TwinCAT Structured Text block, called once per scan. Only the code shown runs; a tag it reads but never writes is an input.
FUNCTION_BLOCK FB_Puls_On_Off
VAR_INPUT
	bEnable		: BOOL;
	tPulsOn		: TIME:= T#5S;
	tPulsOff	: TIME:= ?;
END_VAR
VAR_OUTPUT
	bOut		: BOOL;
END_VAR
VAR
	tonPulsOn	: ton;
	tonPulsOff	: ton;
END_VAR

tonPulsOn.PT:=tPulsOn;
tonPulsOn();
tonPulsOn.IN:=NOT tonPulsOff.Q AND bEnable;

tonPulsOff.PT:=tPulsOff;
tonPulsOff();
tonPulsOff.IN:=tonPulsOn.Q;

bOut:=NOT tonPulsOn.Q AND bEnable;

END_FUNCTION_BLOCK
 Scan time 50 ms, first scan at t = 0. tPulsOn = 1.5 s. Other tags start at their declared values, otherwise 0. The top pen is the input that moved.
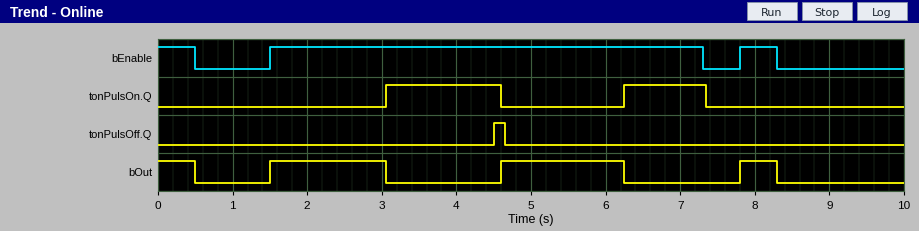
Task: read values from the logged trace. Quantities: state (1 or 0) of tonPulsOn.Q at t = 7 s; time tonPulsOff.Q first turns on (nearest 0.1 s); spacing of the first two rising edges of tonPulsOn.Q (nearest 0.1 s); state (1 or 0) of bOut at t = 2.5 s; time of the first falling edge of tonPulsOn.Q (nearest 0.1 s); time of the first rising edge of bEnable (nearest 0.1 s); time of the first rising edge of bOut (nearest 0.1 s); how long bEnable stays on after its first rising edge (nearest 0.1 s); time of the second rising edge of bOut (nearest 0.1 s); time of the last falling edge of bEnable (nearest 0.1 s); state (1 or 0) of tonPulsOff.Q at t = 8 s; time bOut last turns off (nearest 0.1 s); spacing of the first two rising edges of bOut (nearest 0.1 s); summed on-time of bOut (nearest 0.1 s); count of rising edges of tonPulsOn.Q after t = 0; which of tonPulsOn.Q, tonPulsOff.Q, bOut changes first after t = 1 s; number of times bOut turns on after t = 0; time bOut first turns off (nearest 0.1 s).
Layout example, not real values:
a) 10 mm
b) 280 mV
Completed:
a) 1
b) 4.5 s
c) 3.2 s
d) 1
e) 4.6 s
f) 1.5 s
g) 1.5 s
h) 5.8 s
i) 4.6 s
j) 8.3 s
k) 0
l) 8.3 s
m) 3.1 s
n) 4.2 s
o) 2
p) bOut
q) 3
r) 0.5 s
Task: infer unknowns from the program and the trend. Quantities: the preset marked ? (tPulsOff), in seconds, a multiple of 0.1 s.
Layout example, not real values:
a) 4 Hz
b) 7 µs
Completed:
a) 1.4 s
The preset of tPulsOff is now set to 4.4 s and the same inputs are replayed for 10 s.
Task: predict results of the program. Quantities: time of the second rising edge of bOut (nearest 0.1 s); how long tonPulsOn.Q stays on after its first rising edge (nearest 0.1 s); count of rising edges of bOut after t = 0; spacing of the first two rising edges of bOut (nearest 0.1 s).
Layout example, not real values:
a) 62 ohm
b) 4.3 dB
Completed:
a) 7.8 s
b) 4.3 s
c) 2
d) 6.3 s
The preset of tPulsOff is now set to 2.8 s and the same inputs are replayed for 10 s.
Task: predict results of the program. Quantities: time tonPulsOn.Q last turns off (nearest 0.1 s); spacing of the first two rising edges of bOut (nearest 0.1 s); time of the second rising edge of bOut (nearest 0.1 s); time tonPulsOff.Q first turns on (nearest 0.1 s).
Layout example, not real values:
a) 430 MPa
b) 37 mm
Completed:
a) 6.0 s
b) 4.5 s
c) 6.0 s
d) 5.9 s
